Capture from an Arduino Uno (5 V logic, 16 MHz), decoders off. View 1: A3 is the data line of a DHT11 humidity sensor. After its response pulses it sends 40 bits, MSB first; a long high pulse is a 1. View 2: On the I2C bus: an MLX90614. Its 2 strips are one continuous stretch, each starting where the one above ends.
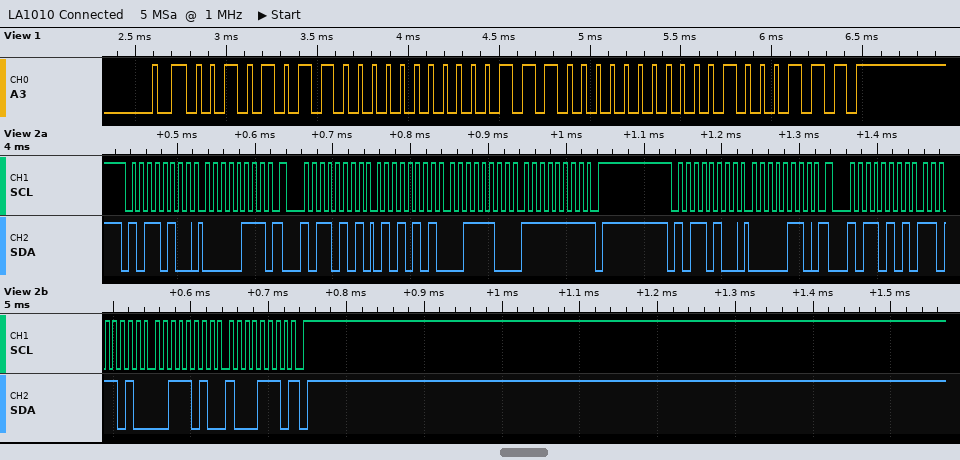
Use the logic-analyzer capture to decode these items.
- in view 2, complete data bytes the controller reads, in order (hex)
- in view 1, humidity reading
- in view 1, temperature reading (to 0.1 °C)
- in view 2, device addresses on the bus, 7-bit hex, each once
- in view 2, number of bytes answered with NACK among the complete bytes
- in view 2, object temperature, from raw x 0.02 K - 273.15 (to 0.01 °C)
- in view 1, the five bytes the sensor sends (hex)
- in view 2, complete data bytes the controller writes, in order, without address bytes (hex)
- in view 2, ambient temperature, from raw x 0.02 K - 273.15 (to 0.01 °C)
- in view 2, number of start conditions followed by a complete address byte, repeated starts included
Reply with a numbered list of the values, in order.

1. 55 3C FF DA 3A 8E
2. 43 %
3. 28.0 °C
4. 0x5A
5. 2
6. 35.75 °C
7. 2B 00 1C 00 47
8. 07 06
9. 28.17 °C
10. 4
